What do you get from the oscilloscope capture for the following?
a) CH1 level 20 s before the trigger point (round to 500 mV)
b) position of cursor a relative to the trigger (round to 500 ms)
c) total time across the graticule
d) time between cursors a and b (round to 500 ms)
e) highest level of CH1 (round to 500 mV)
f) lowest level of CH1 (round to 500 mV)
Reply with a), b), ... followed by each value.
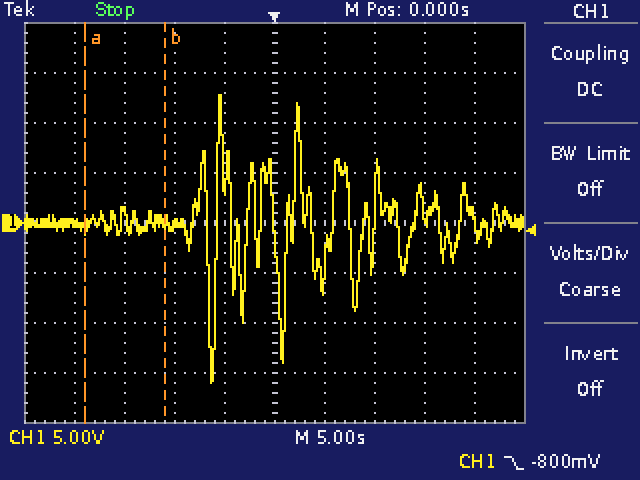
a) 0.0 V
b) -19.0 s
c) 50 s
d) 8.0 s
e) 13.0 V
f) -16.0 V
